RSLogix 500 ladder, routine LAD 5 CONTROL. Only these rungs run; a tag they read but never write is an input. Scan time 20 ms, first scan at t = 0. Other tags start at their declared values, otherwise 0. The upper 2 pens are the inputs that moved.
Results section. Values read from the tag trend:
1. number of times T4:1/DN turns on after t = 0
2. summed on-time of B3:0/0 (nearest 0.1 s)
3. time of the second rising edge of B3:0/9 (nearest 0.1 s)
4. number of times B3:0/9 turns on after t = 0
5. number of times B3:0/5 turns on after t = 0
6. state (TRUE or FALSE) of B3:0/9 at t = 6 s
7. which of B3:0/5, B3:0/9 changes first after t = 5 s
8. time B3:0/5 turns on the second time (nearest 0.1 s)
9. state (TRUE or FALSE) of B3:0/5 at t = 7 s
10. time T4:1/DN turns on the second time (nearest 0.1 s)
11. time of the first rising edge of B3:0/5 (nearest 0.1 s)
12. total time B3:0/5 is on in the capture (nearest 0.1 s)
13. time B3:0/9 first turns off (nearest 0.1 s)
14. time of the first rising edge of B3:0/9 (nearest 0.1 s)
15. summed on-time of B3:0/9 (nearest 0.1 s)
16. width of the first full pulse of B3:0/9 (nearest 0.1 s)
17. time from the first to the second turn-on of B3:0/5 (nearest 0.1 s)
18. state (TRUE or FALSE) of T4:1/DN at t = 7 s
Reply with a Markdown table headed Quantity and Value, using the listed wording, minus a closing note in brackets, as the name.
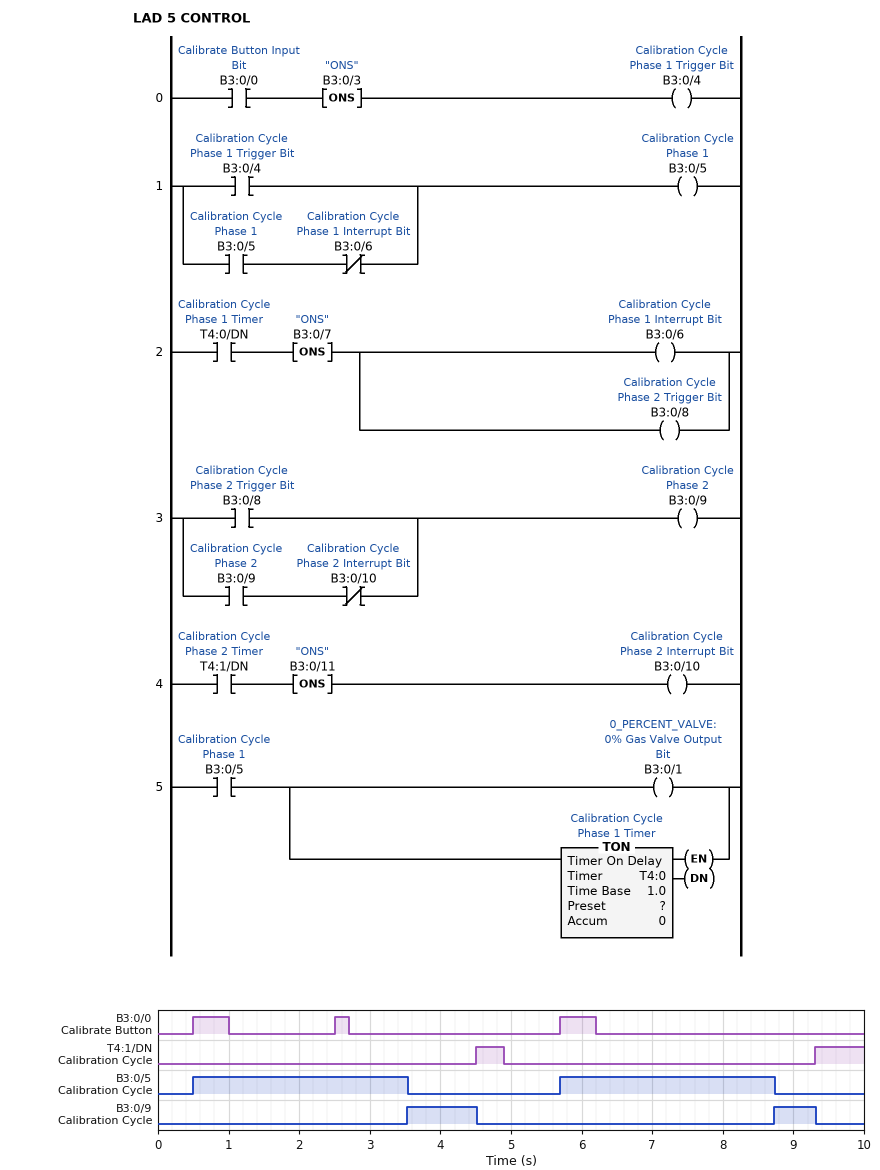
| Quantity | Value |
|---|---|
| number of times T4:1/DN turns on after t = 0 | 2 |
| summed on-time of B3:0/0 | 1.2 s |
| time of the second rising edge of B3:0/9 | 8.7 s |
| number of times B3:0/9 turns on after t = 0 | 2 |
| number of times B3:0/5 turns on after t = 0 | 2 |
| state (TRUE or FALSE) of B3:0/9 at t = 6 s | FALSE |
| which of B3:0/5, B3:0/9 changes first after t = 5 s | B3:0/5 |
| time B3:0/5 turns on the second time | 5.7 s |
| state (TRUE or FALSE) of B3:0/5 at t = 7 s | TRUE |
| time T4:1/DN turns on the second time | 9.3 s |
| time of the first rising edge of B3:0/5 | 0.5 s |
| total time B3:0/5 is on in the capture | 6.1 s |
| time B3:0/9 first turns off | 4.5 s |
| time of the first rising edge of B3:0/9 | 3.5 s |
| summed on-time of B3:0/9 | 1.6 s |
| width of the first full pulse of B3:0/9 | 1.0 s |
| time from the first to the second turn-on of B3:0/5 | 5.2 s |
| state (TRUE or FALSE) of T4:1/DN at t = 7 s | FALSE |
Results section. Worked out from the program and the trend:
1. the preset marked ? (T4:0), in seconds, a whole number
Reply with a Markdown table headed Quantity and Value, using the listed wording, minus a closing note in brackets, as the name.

| Quantity | Value |
|---|---|
| the preset marked ? (T4:0), in seconds, a whole number | 3 s |
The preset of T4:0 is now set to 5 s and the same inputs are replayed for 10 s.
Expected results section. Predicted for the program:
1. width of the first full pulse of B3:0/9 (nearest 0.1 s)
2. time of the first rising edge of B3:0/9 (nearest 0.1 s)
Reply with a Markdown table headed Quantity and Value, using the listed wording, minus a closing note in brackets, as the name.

| Quantity | Value |
|---|---|
| width of the first full pulse of B3:0/9 | 3.8 s |
| time of the first rising edge of B3:0/9 | 5.5 s |
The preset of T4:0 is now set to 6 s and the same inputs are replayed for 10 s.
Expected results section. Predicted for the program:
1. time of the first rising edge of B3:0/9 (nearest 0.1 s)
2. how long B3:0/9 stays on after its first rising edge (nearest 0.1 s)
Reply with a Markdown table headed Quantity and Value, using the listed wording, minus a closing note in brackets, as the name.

| Quantity | Value |
|---|---|
| time of the first rising edge of B3:0/9 | 6.5 s |
| how long B3:0/9 stays on after its first rising edge | 2.8 s |
